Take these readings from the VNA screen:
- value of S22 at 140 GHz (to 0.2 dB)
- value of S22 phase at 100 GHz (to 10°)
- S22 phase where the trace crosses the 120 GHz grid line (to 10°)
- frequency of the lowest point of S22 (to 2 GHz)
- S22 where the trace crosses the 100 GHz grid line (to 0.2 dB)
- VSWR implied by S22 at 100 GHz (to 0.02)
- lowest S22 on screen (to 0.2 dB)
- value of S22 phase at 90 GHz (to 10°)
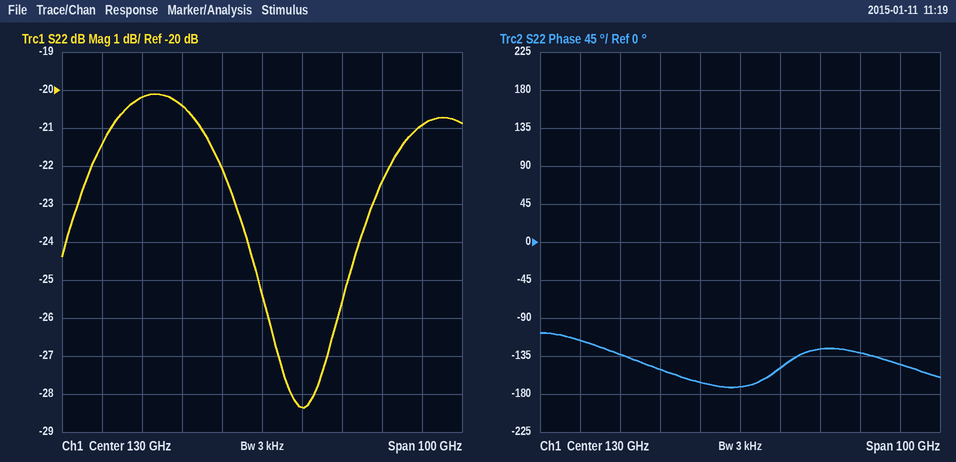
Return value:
-28.4 dB
-130°
-170°
140 GHz
-20.2 dB
1.22
-28.4 dB
-120°
